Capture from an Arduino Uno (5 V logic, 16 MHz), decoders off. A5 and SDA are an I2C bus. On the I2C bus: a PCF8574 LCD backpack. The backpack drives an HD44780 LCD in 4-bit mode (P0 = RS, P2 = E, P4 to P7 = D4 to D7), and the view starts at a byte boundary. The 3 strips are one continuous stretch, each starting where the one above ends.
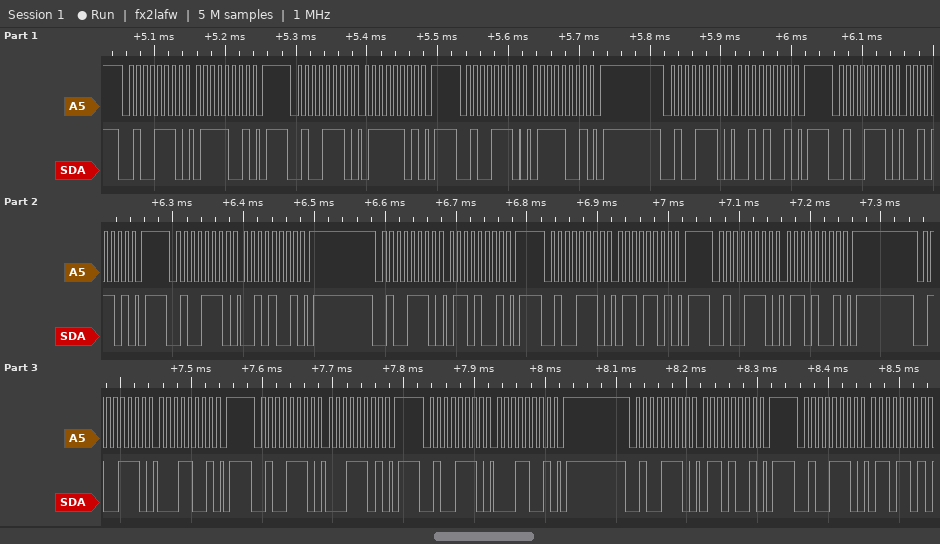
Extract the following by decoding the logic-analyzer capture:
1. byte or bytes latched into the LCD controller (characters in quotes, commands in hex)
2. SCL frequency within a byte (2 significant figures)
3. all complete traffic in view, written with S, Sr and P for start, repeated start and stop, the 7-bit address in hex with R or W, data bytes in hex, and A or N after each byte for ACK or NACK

'r' 'a'
100 kHz
S 27W A 79 A P S 27W A 7D A P S 27W A 79 A P S 27W A 29 A P S 27W A 2D A P S 27W A 29 A P S 27W A 69 A P S 27W A 6D A P S 27W A 69 A P S 27W A 19 A P S 27W A 1D A P S 27W A 19 A P S 27W A 69 A P S 27W A 6D A
